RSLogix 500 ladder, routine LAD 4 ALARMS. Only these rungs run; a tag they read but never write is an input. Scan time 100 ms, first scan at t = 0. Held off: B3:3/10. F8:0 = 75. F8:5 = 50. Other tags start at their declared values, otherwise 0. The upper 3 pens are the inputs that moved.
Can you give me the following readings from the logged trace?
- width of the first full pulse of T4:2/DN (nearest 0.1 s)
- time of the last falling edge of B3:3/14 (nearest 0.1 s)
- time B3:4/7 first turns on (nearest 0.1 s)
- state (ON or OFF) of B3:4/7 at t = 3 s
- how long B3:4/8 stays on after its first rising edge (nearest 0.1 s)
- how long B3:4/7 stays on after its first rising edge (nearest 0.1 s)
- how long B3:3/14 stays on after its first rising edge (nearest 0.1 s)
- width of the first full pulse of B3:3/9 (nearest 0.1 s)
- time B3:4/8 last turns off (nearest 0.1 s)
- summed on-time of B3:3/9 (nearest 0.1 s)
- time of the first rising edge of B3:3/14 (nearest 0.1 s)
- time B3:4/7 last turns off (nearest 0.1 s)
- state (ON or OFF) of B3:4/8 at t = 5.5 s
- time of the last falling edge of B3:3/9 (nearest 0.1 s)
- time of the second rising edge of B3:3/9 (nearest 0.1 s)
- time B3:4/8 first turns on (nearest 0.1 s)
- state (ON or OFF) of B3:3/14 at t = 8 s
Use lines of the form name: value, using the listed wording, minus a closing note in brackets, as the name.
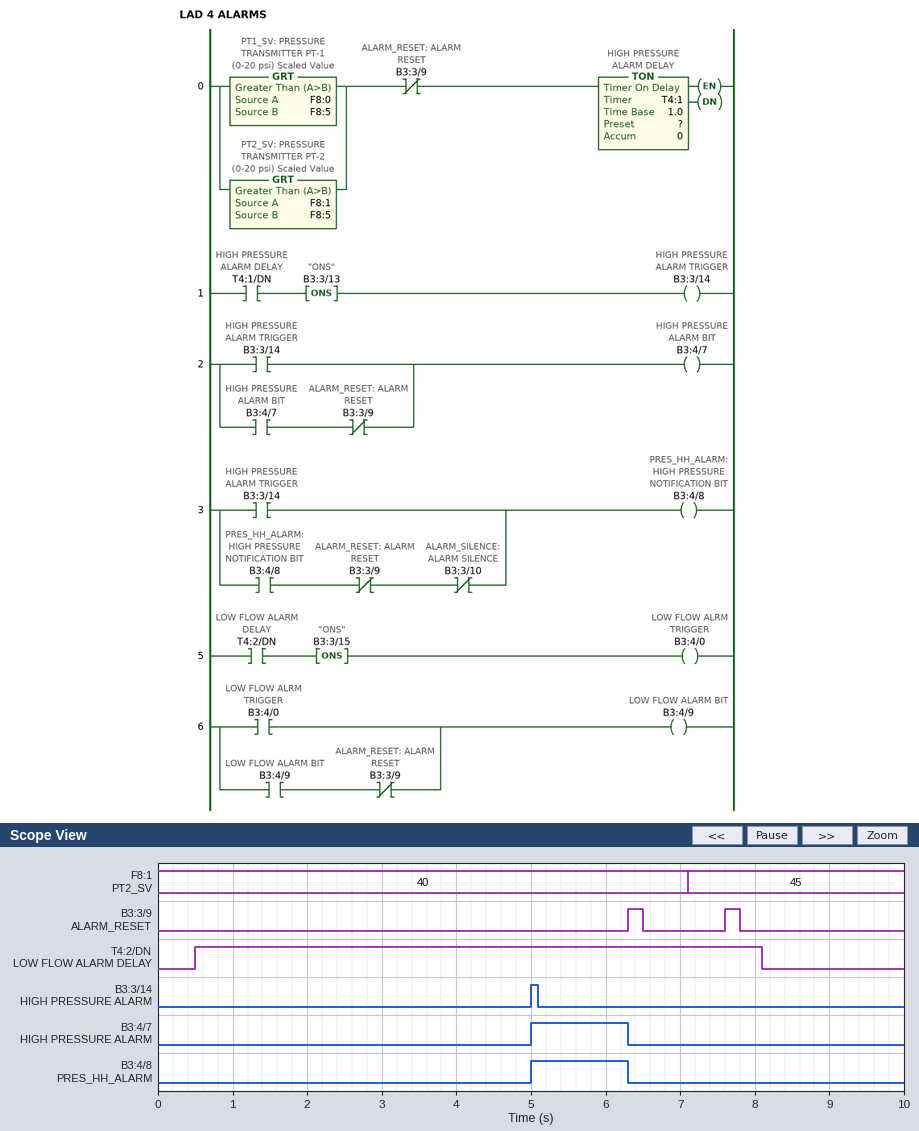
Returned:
width of the first full pulse of T4:2/DN: 7.6 s
time of the last falling edge of B3:3/14: 5.1 s
time B3:4/7 first turns on: 5.0 s
state (ON or OFF) of B3:4/7 at t = 3 s: OFF
how long B3:4/8 stays on after its first rising edge: 1.3 s
how long B3:4/7 stays on after its first rising edge: 1.3 s
how long B3:3/14 stays on after its first rising edge: 0.1 s
width of the first full pulse of B3:3/9: 0.2 s
time B3:4/8 last turns off: 6.3 s
summed on-time of B3:3/9: 0.4 s
time of the first rising edge of B3:3/14: 5.0 s
time B3:4/7 last turns off: 6.3 s
state (ON or OFF) of B3:4/8 at t = 5.5 s: ON
time of the last falling edge of B3:3/9: 7.8 s
time of the second rising edge of B3:3/9: 7.6 s
time B3:4/8 first turns on: 5.0 s
state (ON or OFF) of B3:3/14 at t = 8 s: OFF
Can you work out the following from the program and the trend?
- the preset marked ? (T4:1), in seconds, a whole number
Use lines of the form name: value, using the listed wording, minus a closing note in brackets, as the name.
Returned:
the preset marked ? (T4:1), in seconds, a whole number: 5 s
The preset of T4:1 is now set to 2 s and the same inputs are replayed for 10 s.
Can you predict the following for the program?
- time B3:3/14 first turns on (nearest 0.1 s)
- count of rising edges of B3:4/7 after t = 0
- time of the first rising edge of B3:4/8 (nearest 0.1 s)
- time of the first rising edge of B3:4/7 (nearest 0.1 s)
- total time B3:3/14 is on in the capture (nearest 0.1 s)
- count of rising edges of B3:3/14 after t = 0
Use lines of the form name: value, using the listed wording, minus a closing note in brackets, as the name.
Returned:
time B3:3/14 first turns on: 2.0 s
count of rising edges of B3:4/7 after t = 0: 2
time of the first rising edge of B3:4/8: 2.0 s
time of the first rising edge of B3:4/7: 2.0 s
total time B3:3/14 is on in the capture: 0.2 s
count of rising edges of B3:3/14 after t = 0: 2
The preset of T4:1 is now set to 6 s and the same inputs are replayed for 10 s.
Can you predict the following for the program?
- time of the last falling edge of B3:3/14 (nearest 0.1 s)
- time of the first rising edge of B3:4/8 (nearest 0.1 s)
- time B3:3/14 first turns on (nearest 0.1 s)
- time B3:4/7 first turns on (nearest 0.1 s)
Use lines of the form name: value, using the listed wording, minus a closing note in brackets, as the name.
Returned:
time of the last falling edge of B3:3/14: 6.1 s
time of the first rising edge of B3:4/8: 6.0 s
time B3:3/14 first turns on: 6.0 s
time B3:4/7 first turns on: 6.0 s
